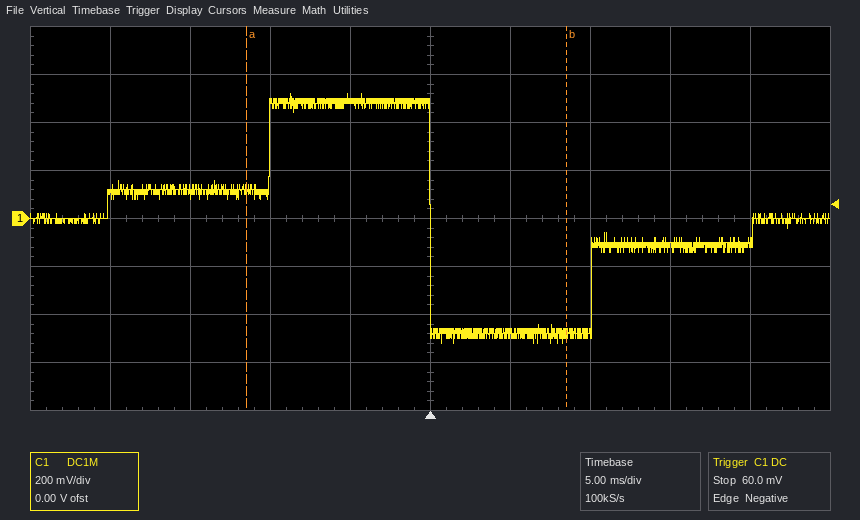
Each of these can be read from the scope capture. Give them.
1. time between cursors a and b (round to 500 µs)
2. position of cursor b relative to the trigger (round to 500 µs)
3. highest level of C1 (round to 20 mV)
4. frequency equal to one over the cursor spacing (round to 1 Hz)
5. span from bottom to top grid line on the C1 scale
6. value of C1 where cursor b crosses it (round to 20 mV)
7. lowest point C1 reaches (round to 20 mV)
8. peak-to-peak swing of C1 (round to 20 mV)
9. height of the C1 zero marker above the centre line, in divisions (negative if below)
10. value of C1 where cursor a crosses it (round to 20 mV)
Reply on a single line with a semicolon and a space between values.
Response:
20.0 ms; +8.5 ms; 520 mV; 50 Hz; 1.6 V; -480 mV; -520 mV; 1.04 V; 0.0 div; 120 mV
